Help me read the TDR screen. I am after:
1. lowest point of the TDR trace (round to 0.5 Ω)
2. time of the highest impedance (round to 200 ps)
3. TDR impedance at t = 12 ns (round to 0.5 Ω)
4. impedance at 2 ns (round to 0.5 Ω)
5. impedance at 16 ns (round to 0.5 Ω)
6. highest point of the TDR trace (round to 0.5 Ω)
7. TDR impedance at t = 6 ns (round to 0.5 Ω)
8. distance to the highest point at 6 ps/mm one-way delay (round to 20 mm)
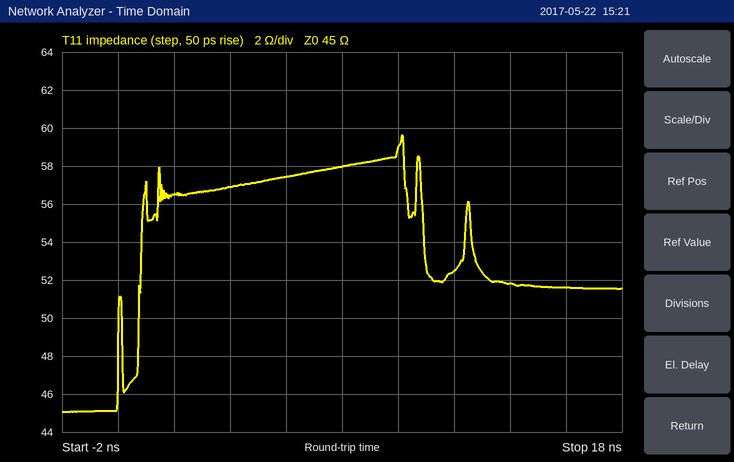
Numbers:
45.0 Ω
10.2 ns
52.5 Ω
56.5 Ω
51.5 Ω
59.5 Ω
57.5 Ω
840 mm
